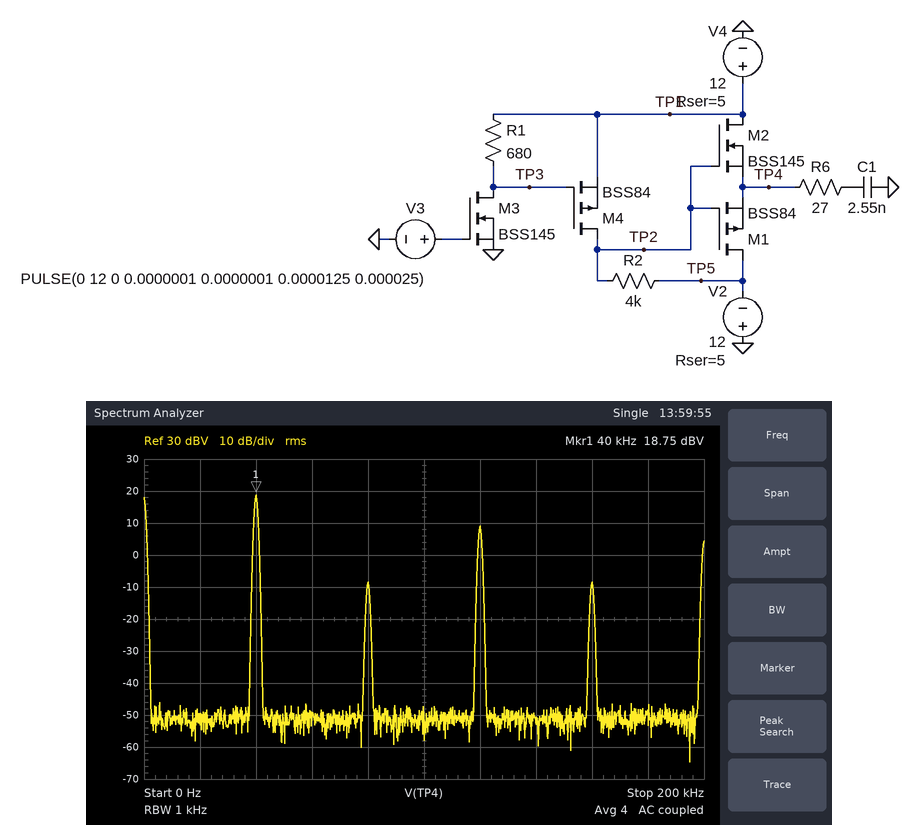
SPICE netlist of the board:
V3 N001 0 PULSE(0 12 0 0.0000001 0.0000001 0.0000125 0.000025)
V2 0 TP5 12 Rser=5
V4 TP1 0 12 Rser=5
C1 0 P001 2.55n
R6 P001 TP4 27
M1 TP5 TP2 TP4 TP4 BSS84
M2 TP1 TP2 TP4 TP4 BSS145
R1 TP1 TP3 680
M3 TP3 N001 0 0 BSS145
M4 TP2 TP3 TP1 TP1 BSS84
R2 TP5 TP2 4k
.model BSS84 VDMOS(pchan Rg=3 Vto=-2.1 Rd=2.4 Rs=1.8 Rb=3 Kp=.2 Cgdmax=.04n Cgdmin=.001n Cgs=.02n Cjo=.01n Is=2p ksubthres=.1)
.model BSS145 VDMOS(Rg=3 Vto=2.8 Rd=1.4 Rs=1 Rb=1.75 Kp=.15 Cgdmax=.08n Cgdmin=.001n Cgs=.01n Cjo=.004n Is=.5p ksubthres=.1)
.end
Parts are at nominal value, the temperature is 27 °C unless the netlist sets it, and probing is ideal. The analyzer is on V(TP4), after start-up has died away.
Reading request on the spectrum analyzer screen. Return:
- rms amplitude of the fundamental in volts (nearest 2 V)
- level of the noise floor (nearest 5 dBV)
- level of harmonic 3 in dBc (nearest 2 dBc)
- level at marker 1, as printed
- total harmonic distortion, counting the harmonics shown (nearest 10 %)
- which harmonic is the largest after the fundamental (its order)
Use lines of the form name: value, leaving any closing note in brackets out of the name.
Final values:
rms amplitude of the fundamental in volts: 8 V
level of the noise floor: -50 dBV
level of harmonic 3 in dBc: -10 dBc
level at marker 1, as printed: 18.75 dBV
total harmonic distortion, counting the harmonics shown: 30 %
which harmonic is the largest after the fundamental: 3
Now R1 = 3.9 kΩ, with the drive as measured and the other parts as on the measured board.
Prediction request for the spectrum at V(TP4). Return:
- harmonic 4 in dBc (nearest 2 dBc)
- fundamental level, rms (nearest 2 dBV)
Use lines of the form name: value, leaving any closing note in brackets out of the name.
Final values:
harmonic 4 in dBc: -20 dBc
fundamental level, rms: 18 dBV
